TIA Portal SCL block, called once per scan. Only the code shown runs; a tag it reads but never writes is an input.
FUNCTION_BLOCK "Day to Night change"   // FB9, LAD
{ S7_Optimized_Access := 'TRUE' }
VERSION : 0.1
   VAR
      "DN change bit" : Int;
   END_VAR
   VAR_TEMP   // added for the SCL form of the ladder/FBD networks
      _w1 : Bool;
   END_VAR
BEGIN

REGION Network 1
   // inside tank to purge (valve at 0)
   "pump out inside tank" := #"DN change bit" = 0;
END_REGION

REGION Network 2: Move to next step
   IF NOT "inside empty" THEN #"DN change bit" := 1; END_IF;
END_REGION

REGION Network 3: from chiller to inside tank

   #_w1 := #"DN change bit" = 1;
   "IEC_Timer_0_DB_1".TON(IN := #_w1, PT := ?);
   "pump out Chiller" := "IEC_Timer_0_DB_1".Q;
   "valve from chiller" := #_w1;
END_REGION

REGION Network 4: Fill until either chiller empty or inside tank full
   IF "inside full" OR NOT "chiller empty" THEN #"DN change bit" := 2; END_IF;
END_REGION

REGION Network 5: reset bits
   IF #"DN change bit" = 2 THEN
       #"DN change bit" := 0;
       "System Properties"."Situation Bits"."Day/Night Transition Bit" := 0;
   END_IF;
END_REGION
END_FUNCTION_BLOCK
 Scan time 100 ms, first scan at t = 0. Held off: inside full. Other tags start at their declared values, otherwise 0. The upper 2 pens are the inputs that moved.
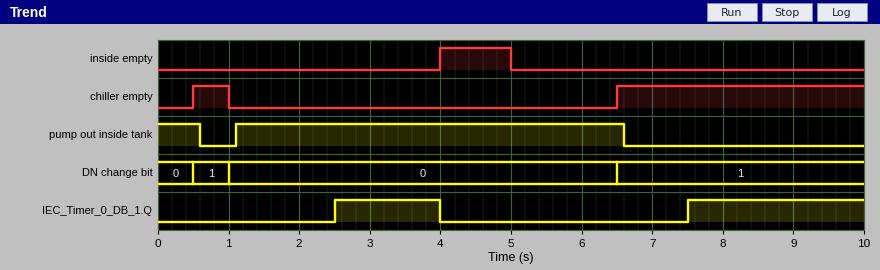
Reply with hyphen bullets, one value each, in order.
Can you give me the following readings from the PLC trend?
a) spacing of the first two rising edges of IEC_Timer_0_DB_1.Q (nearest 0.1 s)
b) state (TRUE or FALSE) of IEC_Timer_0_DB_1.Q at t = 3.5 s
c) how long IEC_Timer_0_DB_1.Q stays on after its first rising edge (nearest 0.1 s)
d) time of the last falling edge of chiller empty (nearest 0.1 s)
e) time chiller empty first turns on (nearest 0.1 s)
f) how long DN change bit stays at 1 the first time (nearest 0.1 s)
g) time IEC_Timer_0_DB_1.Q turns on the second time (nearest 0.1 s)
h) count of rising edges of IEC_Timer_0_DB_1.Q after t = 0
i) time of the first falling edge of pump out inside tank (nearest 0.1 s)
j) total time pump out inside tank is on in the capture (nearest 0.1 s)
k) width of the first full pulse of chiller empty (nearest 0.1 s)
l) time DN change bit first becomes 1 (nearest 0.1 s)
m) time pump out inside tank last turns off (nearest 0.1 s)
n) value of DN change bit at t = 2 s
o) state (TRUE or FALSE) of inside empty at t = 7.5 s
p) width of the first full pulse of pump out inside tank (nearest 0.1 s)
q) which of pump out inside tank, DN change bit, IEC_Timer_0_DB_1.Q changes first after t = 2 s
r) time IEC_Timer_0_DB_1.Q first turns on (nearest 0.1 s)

- 5.0 s
- TRUE
- 1.5 s
- 1.0 s
- 0.5 s
- 0.5 s
- 7.5 s
- 2
- 0.6 s
- 6.1 s
- 0.5 s
- 0.5 s
- 6.6 s
- 0
- FALSE
- 5.5 s
- IEC_Timer_0_DB_1.Q
- 2.5 s
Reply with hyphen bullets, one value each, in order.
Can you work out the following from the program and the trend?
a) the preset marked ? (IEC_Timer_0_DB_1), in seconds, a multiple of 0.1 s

- 2.5 s
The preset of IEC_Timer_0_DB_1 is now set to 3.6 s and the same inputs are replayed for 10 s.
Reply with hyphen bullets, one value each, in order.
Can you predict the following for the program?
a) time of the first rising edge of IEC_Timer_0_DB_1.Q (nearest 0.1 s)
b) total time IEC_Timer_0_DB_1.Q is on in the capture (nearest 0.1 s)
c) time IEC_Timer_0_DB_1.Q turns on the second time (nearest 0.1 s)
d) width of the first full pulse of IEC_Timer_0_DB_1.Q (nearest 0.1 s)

- 3.6 s
- 1.8 s
- 8.6 s
- 0.4 s
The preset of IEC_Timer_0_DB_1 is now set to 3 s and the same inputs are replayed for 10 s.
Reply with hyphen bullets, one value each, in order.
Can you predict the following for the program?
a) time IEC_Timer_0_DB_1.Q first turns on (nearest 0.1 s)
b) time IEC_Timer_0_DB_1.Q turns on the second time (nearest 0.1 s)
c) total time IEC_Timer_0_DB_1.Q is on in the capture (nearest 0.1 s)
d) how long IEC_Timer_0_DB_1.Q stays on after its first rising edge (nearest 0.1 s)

- 3.0 s
- 8.0 s
- 3.0 s
- 1.0 s
